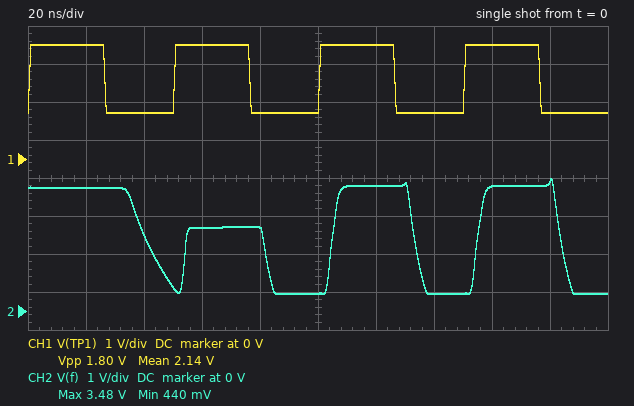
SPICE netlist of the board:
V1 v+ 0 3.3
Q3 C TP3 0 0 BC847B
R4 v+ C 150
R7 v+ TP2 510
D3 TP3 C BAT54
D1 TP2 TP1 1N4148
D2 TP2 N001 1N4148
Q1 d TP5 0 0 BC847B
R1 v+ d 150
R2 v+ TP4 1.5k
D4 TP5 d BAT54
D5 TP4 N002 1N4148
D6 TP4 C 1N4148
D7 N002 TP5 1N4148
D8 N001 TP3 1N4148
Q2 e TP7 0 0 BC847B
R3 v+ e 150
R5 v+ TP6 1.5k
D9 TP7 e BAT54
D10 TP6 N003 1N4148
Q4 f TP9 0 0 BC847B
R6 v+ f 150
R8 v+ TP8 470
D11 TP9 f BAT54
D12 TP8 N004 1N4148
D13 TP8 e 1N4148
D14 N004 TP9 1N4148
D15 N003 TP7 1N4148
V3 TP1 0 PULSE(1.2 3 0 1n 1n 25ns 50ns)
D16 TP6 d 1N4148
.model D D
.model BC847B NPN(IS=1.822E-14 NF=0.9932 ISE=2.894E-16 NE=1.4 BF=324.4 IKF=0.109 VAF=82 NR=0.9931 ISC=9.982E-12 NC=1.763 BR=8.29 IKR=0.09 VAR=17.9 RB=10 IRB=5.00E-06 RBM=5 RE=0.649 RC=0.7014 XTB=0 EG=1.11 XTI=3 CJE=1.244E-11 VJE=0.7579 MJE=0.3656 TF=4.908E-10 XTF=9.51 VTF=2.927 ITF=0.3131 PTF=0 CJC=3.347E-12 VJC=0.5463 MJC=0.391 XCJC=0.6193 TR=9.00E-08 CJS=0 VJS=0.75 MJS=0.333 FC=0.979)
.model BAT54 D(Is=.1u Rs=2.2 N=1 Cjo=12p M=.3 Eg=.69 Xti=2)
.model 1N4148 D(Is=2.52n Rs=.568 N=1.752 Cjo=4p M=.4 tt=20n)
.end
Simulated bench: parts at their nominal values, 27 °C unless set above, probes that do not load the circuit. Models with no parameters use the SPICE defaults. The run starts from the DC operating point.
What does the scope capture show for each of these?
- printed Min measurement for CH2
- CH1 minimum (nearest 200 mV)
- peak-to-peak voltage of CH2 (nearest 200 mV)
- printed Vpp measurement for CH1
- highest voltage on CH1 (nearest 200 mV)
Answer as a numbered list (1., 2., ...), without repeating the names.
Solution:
1. 440 mV
2. 1.2 V
3. 3.0 V
4. 1.80 V
5. 3.0 V
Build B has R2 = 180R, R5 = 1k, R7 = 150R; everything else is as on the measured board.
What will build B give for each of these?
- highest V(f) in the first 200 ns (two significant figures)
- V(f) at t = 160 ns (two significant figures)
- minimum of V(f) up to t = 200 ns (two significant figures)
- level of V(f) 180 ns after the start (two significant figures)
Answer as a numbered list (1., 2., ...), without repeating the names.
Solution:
1. 3.6 V
2. 3.2 V
3. 390 mV
4. 3.3 V
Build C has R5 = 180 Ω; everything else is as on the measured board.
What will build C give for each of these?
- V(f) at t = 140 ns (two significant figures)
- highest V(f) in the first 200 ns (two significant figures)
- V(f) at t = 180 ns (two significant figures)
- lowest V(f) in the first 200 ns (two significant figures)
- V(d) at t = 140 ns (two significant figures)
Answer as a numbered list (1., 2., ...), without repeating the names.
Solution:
1. 460 mV
2. 3.6 V
3. 3.4 V
4. 390 mV
5. 510 mV
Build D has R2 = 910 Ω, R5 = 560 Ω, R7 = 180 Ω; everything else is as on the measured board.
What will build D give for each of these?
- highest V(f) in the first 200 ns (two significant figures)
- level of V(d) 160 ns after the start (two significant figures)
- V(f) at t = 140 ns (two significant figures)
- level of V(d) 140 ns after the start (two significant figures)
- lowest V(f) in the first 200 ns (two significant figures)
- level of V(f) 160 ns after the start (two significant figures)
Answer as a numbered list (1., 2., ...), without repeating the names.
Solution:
1. 3.6 V
2. 2.4 V
3. 450 mV
4. 480 mV
5. 390 mV
6. 3.2 V
